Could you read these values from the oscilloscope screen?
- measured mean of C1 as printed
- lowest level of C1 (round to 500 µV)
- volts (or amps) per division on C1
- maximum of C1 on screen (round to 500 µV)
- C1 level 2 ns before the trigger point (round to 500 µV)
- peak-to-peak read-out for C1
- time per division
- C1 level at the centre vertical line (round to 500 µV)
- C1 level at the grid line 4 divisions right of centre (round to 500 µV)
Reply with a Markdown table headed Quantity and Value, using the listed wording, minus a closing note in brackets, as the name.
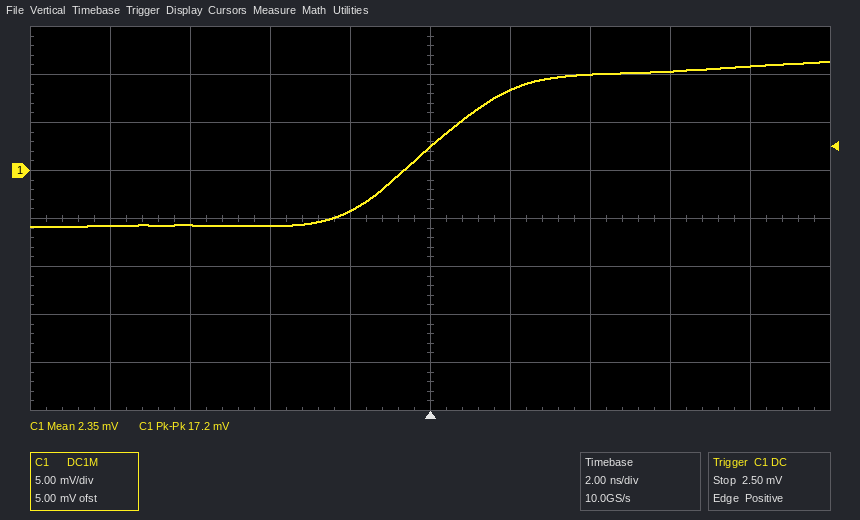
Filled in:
| Quantity | Value |
|---|---|
| measured mean of C1 as printed | 2.35 mV |
| lowest level of C1 | -6.0 mV |
| volts (or amps) per division on C1 | 5 mV |
| maximum of C1 on screen | 11.5 mV |
| C1 level 2 ns before the trigger point | -4.0 mV |
| peak-to-peak read-out for C1 | 17.2 mV |
| time per division | 2 ns |
| C1 level at the centre vertical line | 2.5 mV |
| C1 level at the grid line 4 divisions right of centre | 11.0 mV |
